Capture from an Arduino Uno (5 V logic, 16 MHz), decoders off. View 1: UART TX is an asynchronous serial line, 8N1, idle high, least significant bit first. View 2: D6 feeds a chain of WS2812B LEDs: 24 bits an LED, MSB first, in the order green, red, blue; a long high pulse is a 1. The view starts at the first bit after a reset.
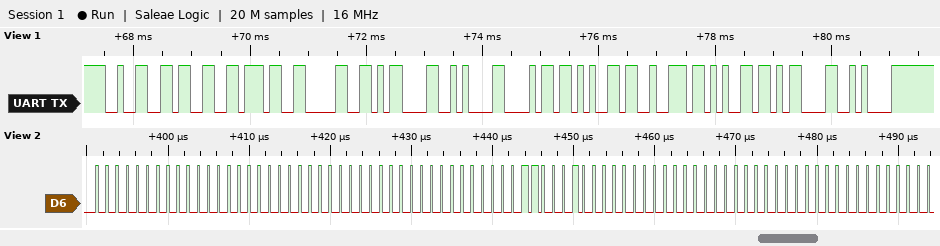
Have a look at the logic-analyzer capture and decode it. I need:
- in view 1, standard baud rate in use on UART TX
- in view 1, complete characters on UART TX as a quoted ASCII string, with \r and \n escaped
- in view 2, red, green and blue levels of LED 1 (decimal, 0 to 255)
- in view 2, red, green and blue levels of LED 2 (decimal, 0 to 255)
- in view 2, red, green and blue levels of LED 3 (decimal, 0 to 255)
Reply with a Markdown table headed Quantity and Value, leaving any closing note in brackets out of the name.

| Quantity | Value |
|---|---|
| in view 1, standard baud rate in use on UART TX | 9600 baud |
| in view 1, complete characters on UART TX as a quoted ASCII string, with \r and \n escaped | "2370\r\nhere\r\n" |
| in view 2, red, green and blue levels of LED 1 | 0, 0, 0 |
| in view 2, red, green and blue levels of LED 2 | 0, 0, 49 |
| in view 2, red, green and blue levels of LED 3 | 0, 0, 0 |
